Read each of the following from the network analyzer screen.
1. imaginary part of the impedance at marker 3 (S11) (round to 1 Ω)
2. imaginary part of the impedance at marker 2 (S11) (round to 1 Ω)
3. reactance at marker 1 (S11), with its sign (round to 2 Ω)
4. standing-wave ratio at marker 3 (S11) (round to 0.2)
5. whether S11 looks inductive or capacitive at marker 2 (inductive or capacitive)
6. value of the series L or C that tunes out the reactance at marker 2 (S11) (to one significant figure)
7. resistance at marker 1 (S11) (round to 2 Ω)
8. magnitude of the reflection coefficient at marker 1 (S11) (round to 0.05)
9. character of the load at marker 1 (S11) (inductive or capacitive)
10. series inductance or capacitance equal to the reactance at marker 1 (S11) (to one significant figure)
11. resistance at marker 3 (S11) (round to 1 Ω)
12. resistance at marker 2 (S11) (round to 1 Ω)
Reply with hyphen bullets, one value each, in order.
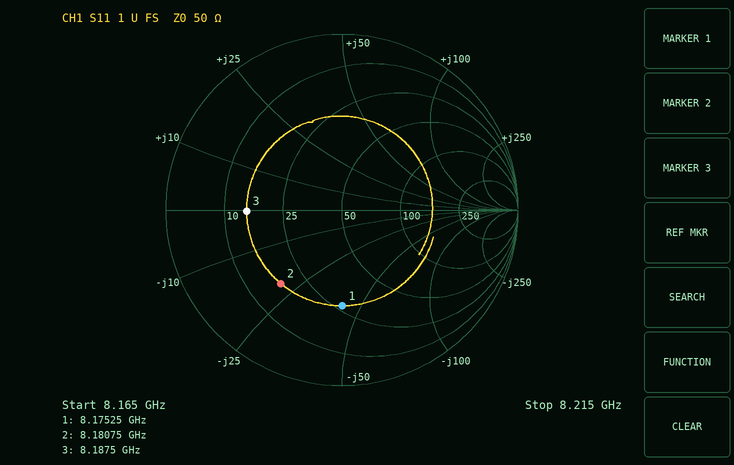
- 0 Ω
- -21 Ω
- -42 Ω
- 3.4
- capacitive
- 400 pH
- 28 Ω
- 0.55
- capacitive
- 500 fF
- 15 Ω
- 18 Ω
